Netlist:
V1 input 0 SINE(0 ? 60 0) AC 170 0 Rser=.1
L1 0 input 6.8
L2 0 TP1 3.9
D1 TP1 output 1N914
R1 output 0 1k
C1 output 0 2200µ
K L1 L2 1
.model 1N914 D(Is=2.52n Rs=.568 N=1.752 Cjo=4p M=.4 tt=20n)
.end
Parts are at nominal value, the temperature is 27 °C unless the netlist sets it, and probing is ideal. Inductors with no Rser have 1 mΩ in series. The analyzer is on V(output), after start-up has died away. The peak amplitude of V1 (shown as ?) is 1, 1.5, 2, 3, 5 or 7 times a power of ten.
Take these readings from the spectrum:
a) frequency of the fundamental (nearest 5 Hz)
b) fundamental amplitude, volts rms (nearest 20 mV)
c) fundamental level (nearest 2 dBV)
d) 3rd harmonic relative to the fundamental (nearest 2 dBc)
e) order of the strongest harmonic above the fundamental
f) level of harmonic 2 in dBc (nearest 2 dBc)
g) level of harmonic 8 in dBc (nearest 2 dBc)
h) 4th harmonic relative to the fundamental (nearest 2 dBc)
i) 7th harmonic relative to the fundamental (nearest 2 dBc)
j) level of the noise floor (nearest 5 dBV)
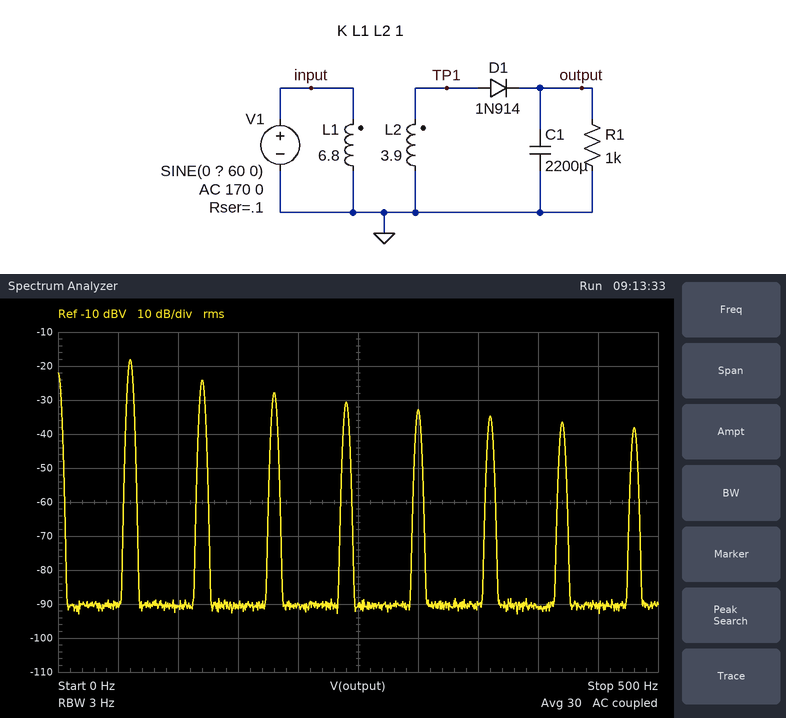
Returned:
60 Hz
120 mV
-18 dBV
-10 dBc
2
-6 dBc
-20 dBc
-12 dBc
-18 dBc
-90 dBV
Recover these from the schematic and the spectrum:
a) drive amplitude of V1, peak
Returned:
100 V
